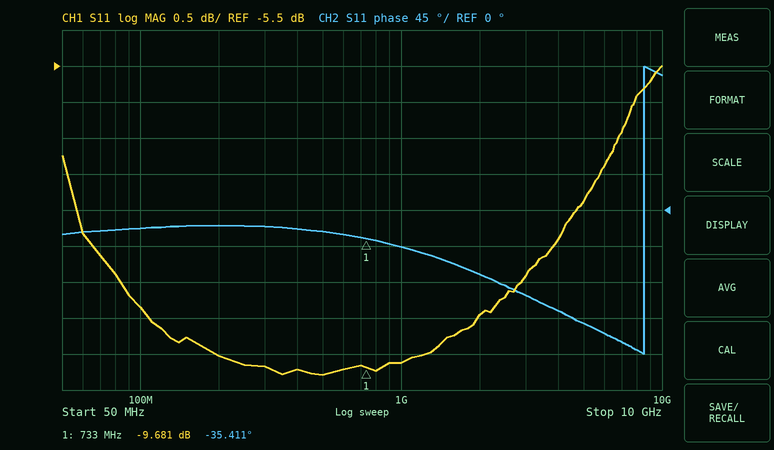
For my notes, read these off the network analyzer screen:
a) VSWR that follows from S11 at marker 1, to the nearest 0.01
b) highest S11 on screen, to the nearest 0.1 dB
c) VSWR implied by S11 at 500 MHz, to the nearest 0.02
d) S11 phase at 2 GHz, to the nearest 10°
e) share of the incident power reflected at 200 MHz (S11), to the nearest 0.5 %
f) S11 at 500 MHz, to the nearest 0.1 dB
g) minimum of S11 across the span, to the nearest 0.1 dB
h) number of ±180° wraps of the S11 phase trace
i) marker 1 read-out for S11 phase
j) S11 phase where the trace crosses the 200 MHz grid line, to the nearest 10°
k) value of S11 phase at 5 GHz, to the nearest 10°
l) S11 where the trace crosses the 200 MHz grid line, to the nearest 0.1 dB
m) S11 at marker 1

1.98
-5.5 dB
1.96
-80°
11.0 %
-9.8 dB
-9.8 dB
1
-35.411°
-20°
-140°
-9.5 dB
-9.681 dB
